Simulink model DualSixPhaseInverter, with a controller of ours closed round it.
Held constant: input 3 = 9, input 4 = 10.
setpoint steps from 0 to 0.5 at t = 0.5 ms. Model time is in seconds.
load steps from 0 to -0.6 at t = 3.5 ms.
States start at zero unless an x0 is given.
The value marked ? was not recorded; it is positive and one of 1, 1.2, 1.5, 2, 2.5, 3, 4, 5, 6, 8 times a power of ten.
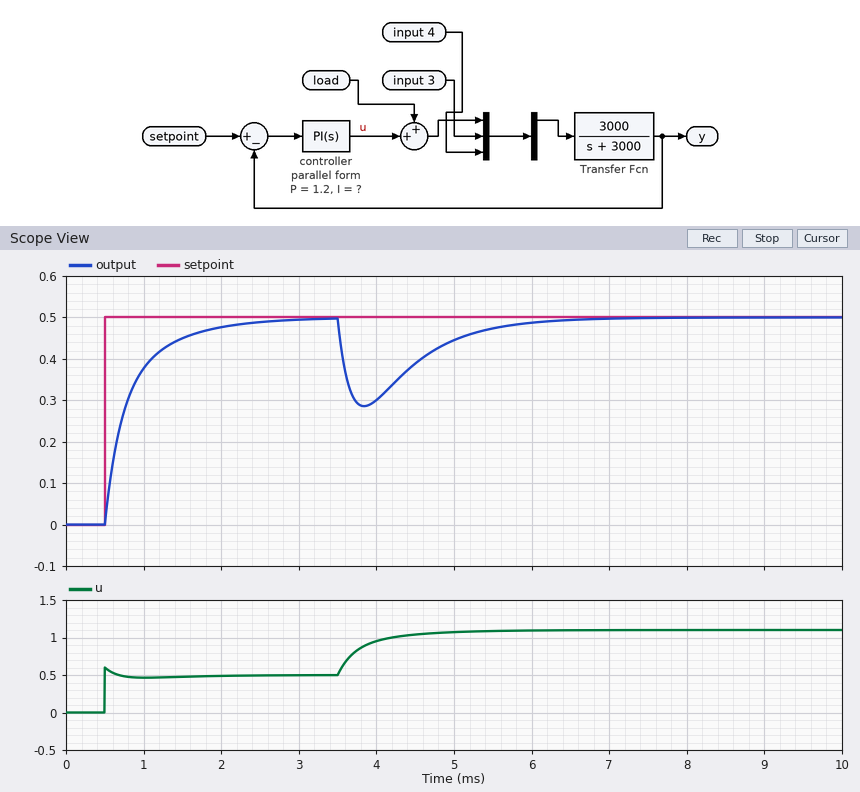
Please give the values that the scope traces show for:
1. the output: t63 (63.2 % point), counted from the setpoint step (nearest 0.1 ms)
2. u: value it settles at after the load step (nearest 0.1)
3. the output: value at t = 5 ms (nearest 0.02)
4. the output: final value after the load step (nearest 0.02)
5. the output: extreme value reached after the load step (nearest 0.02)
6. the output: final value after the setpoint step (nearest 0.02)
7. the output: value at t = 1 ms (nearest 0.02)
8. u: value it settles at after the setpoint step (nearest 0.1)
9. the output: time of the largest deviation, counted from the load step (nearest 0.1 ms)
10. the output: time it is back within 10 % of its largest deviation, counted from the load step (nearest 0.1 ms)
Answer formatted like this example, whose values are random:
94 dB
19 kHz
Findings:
0.3 ms
1.1
0.44
0.50
0.28
0.50
0.38
0.5
0.3 ms
2.2 ms
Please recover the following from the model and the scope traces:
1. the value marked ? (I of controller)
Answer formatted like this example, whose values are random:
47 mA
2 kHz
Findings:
2500
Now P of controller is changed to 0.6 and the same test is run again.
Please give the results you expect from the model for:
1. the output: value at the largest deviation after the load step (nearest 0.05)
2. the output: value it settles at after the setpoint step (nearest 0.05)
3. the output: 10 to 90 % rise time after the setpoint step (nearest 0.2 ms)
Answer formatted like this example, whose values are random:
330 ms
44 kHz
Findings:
0.25
0.50
0.8 ms
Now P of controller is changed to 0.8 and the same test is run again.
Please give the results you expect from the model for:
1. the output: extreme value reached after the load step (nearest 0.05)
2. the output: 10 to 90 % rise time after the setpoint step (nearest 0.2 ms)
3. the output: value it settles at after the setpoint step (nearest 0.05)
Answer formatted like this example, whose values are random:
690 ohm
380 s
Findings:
0.25
0.8 ms
0.50
